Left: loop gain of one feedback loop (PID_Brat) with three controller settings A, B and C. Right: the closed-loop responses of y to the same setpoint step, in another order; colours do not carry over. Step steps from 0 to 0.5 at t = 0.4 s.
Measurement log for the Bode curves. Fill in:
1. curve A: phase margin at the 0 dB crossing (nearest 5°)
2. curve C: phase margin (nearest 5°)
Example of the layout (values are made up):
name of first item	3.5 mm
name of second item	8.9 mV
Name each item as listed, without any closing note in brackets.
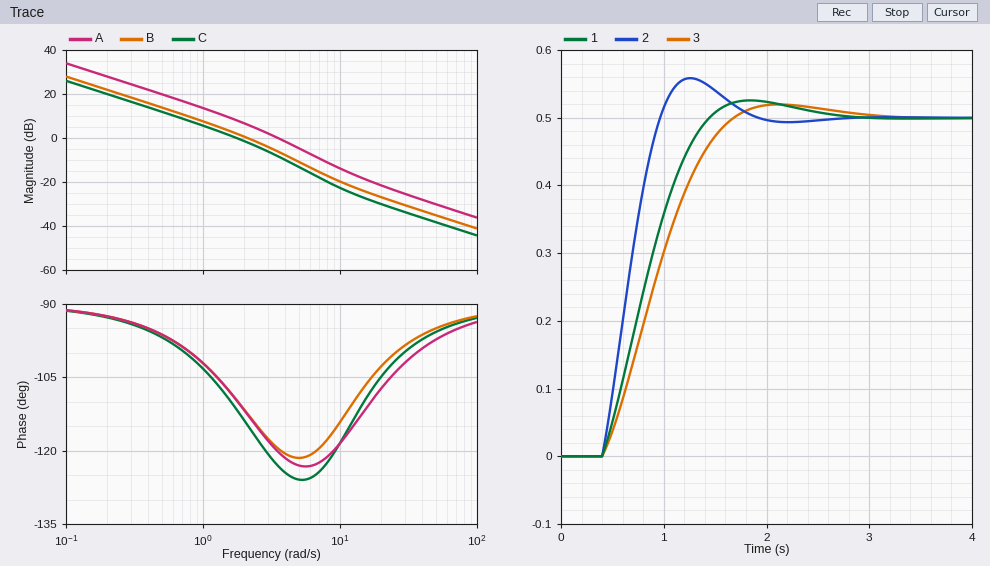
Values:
curve A: phase margin at the 0 dB crossing	60°
curve C: phase margin	70°
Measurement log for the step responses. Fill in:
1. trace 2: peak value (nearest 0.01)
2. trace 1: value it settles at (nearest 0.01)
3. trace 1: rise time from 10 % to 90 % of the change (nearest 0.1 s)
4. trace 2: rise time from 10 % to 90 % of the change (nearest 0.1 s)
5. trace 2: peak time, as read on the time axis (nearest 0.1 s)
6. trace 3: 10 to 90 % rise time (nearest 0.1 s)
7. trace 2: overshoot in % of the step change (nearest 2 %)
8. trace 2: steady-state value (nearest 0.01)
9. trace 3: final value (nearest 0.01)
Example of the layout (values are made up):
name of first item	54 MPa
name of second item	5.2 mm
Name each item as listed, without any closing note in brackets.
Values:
trace 2: peak value	0.56
trace 1: value it settles at	0.50
trace 1: rise time from 10 % to 90 % of the change	0.7 s
trace 2: rise time from 10 % to 90 % of the change	0.4 s
trace 2: peak time, as read on the time axis	1.3 s
trace 3: 10 to 90 % rise time	0.9 s
trace 2: overshoot in % of the step change	12 %
trace 2: steady-state value	0.50
trace 3: final value	0.50
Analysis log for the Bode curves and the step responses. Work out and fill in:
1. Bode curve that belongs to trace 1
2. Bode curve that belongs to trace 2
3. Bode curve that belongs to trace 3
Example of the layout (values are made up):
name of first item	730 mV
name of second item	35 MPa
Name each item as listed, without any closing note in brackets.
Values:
Bode curve that belongs to trace 1	B
Bode curve that belongs to trace 2	A
Bode curve that belongs to trace 3	C
